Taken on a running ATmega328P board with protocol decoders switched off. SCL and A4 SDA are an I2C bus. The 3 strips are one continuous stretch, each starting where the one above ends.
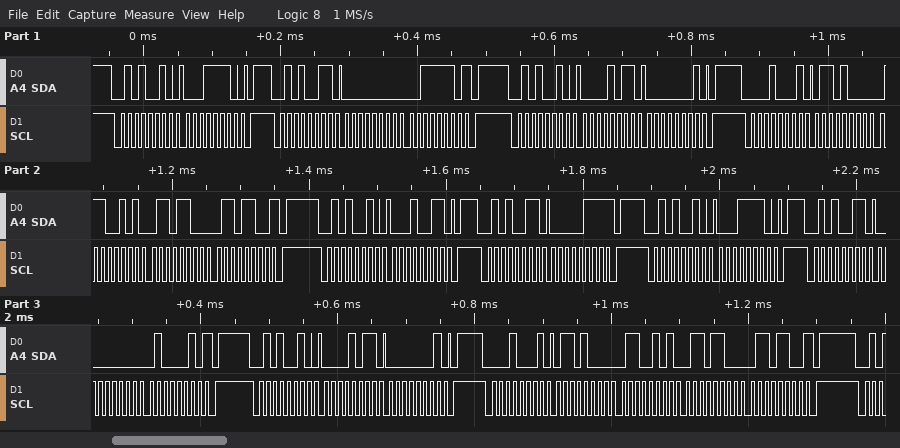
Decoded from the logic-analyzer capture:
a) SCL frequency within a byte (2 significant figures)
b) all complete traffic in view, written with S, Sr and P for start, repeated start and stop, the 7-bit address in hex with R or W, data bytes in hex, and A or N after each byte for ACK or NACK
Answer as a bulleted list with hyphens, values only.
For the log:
- 100 kHz
- S 29W A 1E A P S 29R A 00 A 3E N P S 29W A 0B A 01 A P S 08R A 68 A 65 A 6C A 6C N P S 29W A 13 A P S 29R A 07 N P S 29W A 1E A P S 29R A 00 A 42 N P S 29W A 0B A 01 A P S 08R A 68 A 65 A 6C A 6C N P
